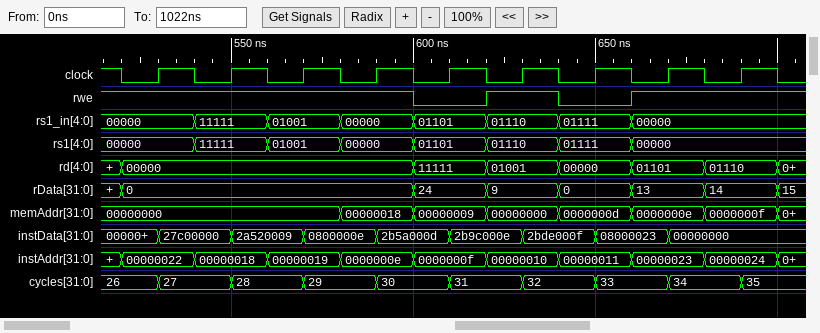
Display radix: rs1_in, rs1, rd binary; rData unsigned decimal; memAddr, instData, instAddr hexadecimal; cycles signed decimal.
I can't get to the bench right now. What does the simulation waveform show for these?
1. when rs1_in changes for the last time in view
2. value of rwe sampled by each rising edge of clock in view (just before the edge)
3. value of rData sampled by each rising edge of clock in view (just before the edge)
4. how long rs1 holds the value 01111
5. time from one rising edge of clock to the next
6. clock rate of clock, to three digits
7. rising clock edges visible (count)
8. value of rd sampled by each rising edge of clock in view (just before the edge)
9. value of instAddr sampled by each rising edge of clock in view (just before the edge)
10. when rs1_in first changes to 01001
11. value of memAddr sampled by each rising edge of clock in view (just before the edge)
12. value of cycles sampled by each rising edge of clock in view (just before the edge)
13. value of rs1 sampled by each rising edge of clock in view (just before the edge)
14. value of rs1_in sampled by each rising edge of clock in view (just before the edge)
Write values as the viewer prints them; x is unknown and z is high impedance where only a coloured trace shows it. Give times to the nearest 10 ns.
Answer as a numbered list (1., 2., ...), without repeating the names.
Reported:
1. 660 ns
2. 1 1 1 1 0 1 0 1 1
3. 0, 0, 0, 0, 24, 9, 0, 13, 14
4. 20 ns
5. 20 ns
6. 50.0 MHz
7. 9
8. 00000, 00000, 00000, 00000, 11111, 01001, 00000, 01101, 01110
9. 00000022, 00000018, 00000019, 0000000e, 0000000f, 00000010, 00000011, 00000023, 00000024
10. 560 ns
11. 00000000, 00000000, 00000000, 00000018, 00000009, 00000000, 0000000d, 0000000e, 0000000f
12. 26, 27, 28, 29, 30, 31, 32, 33, 34
13. 00000, 11111, 01001, 00000, 01101, 01110, 01111, 00000, 00000
14. 00000, 11111, 01001, 00000, 01101, 01110, 01111, 00000, 00000
